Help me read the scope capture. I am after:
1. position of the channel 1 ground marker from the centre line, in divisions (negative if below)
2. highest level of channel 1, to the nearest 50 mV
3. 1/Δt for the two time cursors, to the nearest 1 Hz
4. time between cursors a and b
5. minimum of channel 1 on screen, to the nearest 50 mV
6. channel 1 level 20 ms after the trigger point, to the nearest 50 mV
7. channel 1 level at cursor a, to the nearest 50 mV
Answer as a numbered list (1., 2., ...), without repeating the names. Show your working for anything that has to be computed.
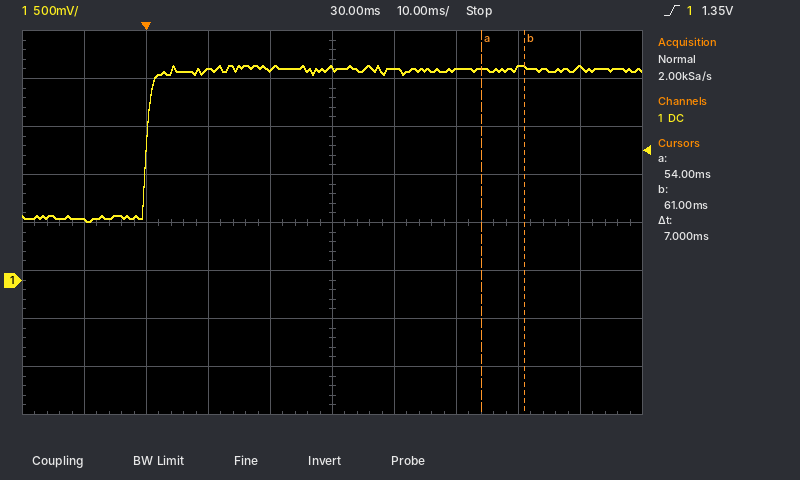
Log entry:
1. -1.2 div
2. 2.25 V
3. 1 / 7 ms ≈ 143 Hz
4. 7 ms
5. 600 mV
6. 2.20 V
7. 2.20 V
